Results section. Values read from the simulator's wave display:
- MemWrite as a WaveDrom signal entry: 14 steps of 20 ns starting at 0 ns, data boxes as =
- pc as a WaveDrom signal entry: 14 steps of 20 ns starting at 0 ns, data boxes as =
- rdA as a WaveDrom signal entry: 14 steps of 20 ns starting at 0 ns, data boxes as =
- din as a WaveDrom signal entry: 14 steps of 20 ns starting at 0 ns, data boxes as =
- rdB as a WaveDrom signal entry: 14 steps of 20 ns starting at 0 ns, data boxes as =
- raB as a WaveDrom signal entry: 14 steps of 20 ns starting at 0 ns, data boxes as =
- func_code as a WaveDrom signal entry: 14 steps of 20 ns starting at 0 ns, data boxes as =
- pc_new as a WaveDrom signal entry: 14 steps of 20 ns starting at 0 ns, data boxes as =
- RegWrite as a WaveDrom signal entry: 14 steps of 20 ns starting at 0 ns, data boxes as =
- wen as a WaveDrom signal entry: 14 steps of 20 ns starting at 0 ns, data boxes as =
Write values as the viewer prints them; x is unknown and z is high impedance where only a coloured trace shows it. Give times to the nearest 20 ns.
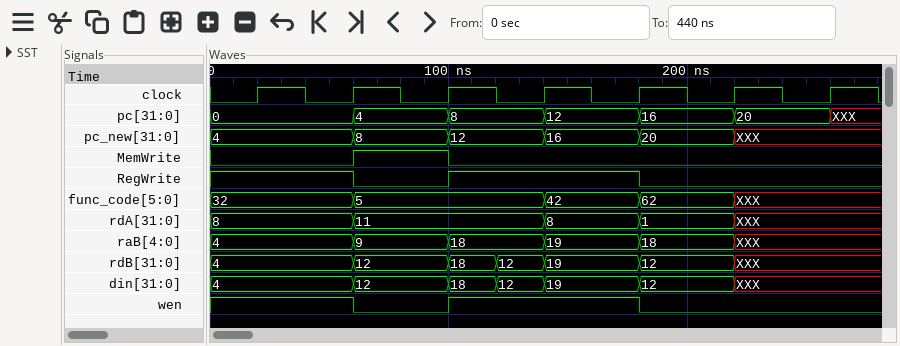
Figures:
{name: 'MemWrite', wave: '0..1.0........'}
{name: 'pc', wave: '=..=.=.=.=.=.x', data: '0 4 8 12 16 20'}
{name: 'rdA', wave: '=..=...=.=.x..', data: '8 11 8 1'}
{name: 'din', wave: '=..=.===.=.x..', data: '4 12 18 12 19 12'}
{name: 'rdB', wave: '=..=.===.=.x..', data: '4 12 18 12 19 12'}
{name: 'raB', wave: '=..=.=.=.=.x..', data: '4 9 18 19 18'}
{name: 'func_code', wave: '=..=...=.=.x..', data: '32 5 42 62'}
{name: 'pc_new', wave: '=..=.=.=.=.x..', data: '4 8 12 16 20'}
{name: 'RegWrite', wave: '1..0.1...0....'}
{name: 'wen', wave: '1..0.1...0....'}
